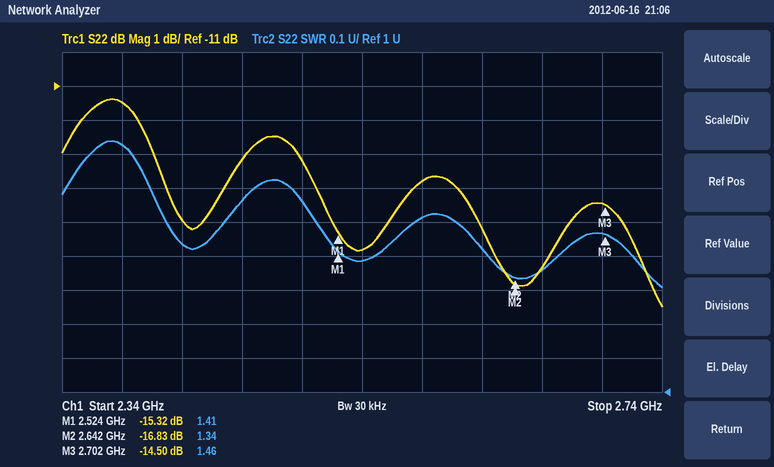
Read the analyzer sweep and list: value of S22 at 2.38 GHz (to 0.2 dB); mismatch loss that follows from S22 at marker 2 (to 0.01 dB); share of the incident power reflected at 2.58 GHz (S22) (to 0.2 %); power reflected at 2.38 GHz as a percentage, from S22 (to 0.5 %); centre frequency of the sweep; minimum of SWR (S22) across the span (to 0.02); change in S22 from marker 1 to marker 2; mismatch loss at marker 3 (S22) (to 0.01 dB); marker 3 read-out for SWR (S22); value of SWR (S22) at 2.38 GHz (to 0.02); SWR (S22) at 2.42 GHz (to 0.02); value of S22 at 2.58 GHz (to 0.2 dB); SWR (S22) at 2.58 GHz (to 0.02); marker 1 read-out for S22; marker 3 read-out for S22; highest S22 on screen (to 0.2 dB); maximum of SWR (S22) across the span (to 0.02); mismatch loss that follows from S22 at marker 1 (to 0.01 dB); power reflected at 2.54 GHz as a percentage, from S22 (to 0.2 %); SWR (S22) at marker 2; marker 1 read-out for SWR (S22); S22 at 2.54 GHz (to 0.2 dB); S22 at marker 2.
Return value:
-11.4 dB
0.09 dB
4.2 %
7.0 %
2.54 GHz
1.30
-1.51 dB
0.16 dB
1.46
1.72
1.44
-13.8 dB
1.52
-15.32 dB
-14.50 dB
-11.4 dB
1.74
0.13 dB
2.6 %
1.34
1.41
-15.8 dB
-16.83 dB
